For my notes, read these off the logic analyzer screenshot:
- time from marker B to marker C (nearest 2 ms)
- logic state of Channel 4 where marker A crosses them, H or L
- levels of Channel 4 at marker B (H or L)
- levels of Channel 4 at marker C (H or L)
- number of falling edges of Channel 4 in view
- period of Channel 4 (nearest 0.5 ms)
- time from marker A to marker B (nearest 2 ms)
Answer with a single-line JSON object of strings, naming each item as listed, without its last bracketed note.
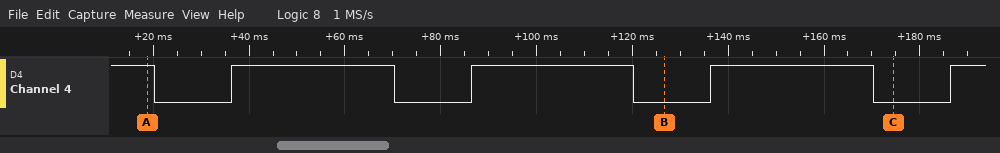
{"time from marker B to marker C": "48 ms", "logic state of Channel 4 where marker A crosses them, H or L": "Channel 4=H", "levels of Channel 4 at marker B": "Channel 4=L", "levels of Channel 4 at marker C": "Channel 4=L", "number of falling edges of Channel 4 in view": "4", "period of Channel 4": "50 ms", "time from marker A to marker B": "108 ms"}
